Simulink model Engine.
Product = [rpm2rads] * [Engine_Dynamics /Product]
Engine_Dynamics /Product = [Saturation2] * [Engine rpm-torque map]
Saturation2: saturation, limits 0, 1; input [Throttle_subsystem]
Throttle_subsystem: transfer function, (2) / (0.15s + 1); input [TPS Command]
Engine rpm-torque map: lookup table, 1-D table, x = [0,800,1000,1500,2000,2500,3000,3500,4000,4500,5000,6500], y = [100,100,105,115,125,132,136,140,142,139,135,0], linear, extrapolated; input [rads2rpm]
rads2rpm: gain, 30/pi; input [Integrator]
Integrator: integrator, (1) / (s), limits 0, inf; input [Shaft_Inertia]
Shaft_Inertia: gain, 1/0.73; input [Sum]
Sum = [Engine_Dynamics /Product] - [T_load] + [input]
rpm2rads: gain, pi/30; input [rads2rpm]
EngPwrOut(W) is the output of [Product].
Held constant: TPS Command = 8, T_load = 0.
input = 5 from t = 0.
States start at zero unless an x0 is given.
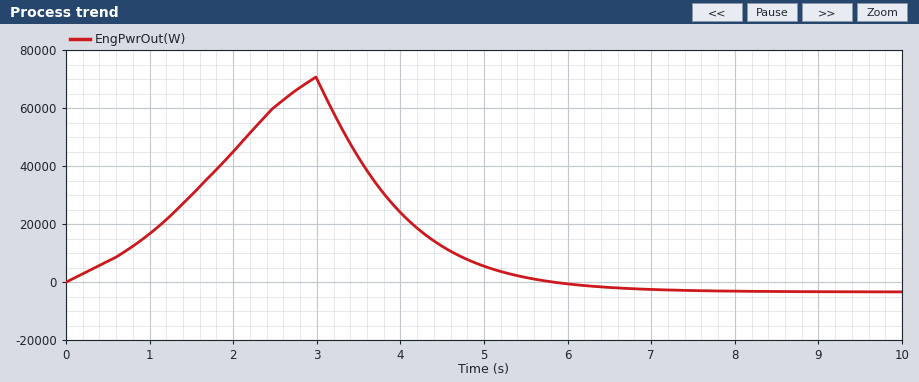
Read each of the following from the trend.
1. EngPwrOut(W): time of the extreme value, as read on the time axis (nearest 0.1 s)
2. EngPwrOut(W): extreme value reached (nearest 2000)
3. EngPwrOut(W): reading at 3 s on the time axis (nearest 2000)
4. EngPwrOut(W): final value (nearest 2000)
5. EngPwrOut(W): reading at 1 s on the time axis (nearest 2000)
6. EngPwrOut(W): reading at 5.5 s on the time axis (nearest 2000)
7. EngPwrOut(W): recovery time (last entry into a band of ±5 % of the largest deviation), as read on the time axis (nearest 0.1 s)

3.0 s
70000
70000
-4000
16000
2000
5.8 s
